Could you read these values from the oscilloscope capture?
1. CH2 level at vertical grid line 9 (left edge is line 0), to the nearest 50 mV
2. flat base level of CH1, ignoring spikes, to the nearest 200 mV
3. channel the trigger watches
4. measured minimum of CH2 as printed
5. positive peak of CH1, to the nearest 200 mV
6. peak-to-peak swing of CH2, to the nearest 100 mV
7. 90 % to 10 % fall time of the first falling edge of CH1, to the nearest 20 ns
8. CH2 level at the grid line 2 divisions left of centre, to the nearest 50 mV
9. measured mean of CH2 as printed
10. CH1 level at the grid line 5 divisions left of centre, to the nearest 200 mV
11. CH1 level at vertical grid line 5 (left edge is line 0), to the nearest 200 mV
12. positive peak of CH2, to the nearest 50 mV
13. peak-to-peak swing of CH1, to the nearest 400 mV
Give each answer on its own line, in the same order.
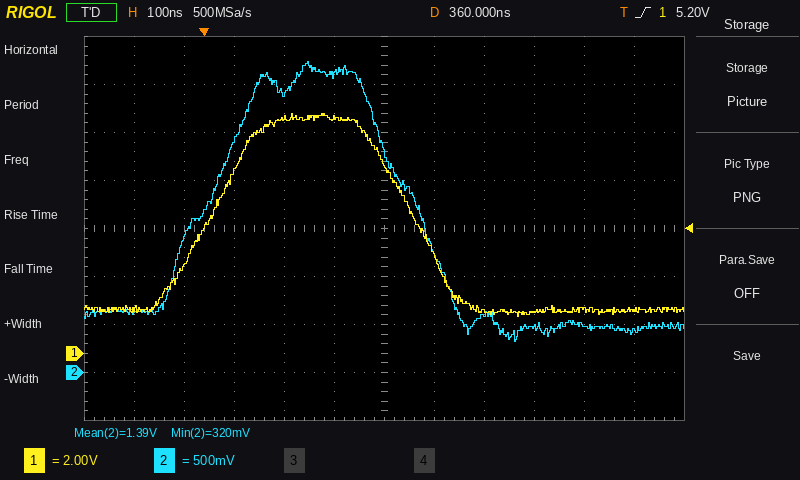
450 mV
1.8 V
CH1
320 mV
10.0 V
2.90 V
160 ns
2.90 V
1.39 V
1.8 V
9.8 V
3.25 V
8.4 V
